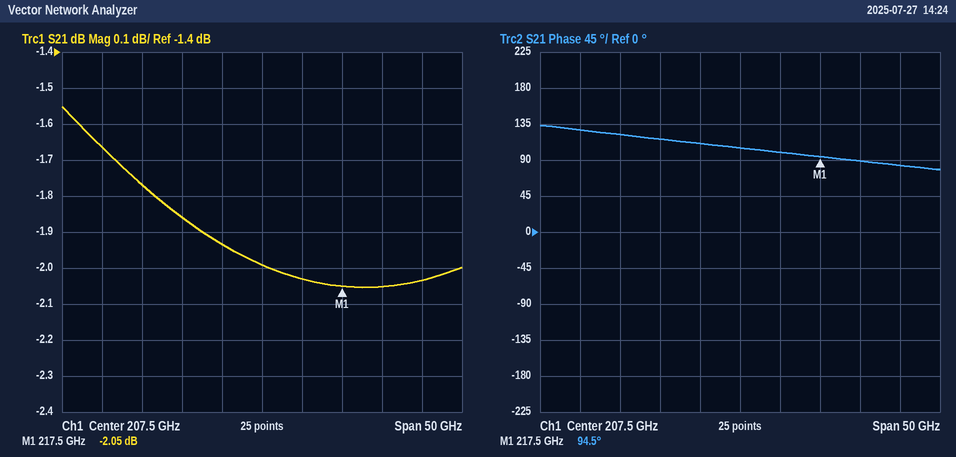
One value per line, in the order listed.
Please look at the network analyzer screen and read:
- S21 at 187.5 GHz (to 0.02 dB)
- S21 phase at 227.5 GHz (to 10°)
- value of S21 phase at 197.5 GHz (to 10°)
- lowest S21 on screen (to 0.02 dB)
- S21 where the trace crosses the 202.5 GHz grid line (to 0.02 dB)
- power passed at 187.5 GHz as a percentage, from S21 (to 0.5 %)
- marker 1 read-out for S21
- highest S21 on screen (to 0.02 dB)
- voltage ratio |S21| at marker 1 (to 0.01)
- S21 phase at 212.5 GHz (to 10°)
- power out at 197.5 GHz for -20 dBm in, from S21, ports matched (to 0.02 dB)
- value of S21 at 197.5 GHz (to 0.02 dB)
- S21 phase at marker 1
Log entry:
-1.66 dB
80°
120°
-2.06 dB
-1.94 dB
68.0 %
-2.05 dB
-1.56 dB
0.79
100°
-21.86 dBm
-1.86 dB
94.5°
